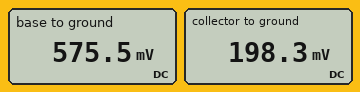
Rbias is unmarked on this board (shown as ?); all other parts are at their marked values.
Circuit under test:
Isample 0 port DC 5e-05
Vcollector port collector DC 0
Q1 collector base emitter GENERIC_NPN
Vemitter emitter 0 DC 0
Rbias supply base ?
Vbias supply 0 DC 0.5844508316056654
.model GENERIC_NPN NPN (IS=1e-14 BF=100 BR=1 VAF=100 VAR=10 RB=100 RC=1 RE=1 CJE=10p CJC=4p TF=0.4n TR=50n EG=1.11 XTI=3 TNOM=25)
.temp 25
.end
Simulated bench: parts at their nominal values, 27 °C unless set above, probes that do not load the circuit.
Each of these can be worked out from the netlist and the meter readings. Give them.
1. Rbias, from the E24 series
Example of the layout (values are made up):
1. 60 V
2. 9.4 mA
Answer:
1. 16 kΩ
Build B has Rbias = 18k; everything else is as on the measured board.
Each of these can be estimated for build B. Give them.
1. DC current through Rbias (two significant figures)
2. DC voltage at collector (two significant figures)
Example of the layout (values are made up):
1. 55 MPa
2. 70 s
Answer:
1. 520 nA
2. 1.9 V
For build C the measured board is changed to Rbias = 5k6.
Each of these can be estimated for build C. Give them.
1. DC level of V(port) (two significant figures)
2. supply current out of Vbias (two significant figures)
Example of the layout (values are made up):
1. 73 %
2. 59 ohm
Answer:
1. 110 mV
2. 1.4 µA
